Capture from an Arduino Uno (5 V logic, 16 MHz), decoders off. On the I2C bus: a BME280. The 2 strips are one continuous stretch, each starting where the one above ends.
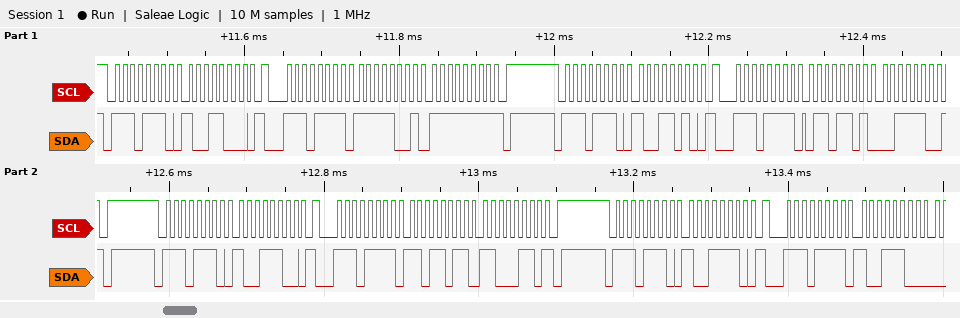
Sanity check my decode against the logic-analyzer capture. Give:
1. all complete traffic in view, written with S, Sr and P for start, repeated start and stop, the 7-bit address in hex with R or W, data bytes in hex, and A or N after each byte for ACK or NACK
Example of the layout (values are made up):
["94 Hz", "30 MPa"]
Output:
["S 77W A 98 A Sr 77R A F9 A FF N P S 77W A 9A A Sr 77R A 6D A 3C N P S 77W A 9C A Sr 77R A DB A C6 N P S 77W A 9E A Sr 77R A 9C A"]
